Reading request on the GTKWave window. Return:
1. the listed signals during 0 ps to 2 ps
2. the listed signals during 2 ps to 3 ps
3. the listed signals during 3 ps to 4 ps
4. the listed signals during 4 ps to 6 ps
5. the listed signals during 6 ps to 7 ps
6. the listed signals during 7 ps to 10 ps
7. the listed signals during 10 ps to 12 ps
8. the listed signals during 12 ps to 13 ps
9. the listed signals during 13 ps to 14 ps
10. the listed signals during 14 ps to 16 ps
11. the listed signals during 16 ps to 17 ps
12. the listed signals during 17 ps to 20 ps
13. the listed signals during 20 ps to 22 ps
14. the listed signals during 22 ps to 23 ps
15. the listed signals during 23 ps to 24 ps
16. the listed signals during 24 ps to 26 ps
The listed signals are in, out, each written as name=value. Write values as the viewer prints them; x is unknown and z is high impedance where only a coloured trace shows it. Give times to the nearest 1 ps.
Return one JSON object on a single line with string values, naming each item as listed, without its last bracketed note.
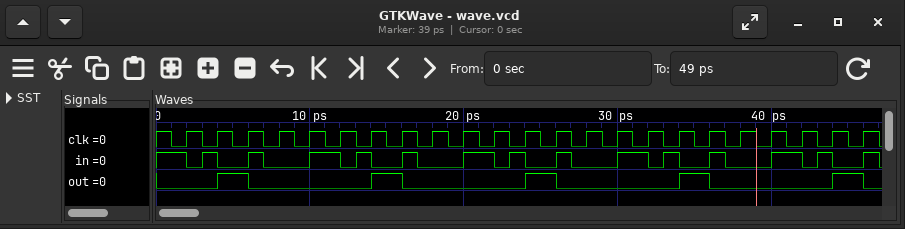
{"the listed signals during 0 ps to 2 ps": "in=1, out=0", "the listed signals during 2 ps to 3 ps": "in=0, out=0", "the listed signals during 3 ps to 4 ps": "in=1, out=0", "the listed signals during 4 ps to 6 ps": "in=0, out=1", "the listed signals during 6 ps to 7 ps": "in=1, out=0", "the listed signals during 7 ps to 10 ps": "in=0, out=0", "the listed signals during 10 ps to 12 ps": "in=1, out=0", "the listed signals during 12 ps to 13 ps": "in=0, out=0", "the listed signals during 13 ps to 14 ps": "in=1, out=0", "the listed signals during 14 ps to 16 ps": "in=0, out=1", "the listed signals during 16 ps to 17 ps": "in=1, out=0", "the listed signals during 17 ps to 20 ps": "in=0, out=0", "the listed signals during 20 ps to 22 ps": "in=1, out=0", "the listed signals during 22 ps to 23 ps": "in=0, out=0", "the listed signals during 23 ps to 24 ps": "in=1, out=0", "the listed signals during 24 ps to 26 ps": "in=0, out=1"}
